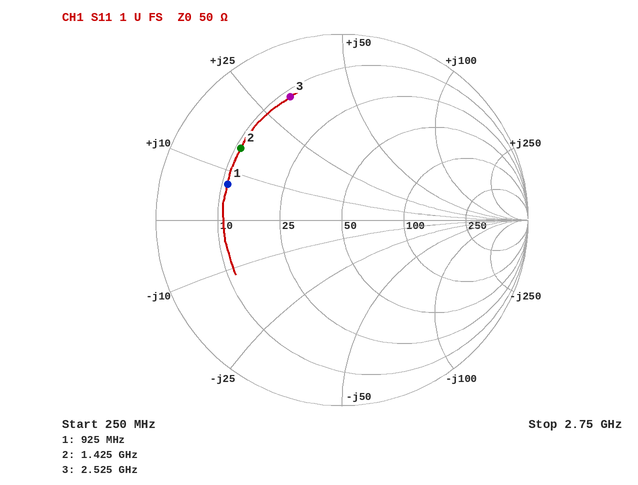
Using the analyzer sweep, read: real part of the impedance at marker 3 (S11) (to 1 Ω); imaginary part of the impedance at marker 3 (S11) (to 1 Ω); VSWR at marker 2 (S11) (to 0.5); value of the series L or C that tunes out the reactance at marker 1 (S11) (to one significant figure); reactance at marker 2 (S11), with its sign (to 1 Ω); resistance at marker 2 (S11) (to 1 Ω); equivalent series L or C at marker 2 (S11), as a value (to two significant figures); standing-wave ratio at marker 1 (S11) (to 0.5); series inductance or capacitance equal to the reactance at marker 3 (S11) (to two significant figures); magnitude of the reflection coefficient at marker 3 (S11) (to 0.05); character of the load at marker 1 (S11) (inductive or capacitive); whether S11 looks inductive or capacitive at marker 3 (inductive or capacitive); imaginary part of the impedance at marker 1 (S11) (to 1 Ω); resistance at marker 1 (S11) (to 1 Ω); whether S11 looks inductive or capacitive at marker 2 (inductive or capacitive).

12 Ω
+32 Ω
5.0
20 pF
+15 Ω
11 Ω
1.7 nH
4.5
2.0 nH
0.70
inductive
inductive
+7 Ω
11 Ω
inductive
